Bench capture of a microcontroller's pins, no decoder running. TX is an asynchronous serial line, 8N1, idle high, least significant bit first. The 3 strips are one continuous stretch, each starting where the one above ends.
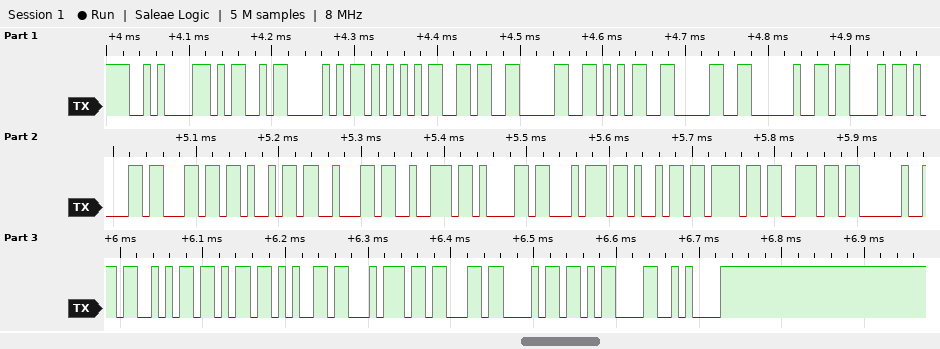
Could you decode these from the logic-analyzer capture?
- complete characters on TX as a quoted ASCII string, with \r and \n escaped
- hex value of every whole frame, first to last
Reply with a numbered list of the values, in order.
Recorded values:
1. "\nMPU6050 Calibration Sketch\r\n"
2. 0A 4D 50 55 36 30 35 30 20 43 61 6C 69 62 72 61 74 69 6F 6E 20 53 6B 65 74 63 68 0D 0A
